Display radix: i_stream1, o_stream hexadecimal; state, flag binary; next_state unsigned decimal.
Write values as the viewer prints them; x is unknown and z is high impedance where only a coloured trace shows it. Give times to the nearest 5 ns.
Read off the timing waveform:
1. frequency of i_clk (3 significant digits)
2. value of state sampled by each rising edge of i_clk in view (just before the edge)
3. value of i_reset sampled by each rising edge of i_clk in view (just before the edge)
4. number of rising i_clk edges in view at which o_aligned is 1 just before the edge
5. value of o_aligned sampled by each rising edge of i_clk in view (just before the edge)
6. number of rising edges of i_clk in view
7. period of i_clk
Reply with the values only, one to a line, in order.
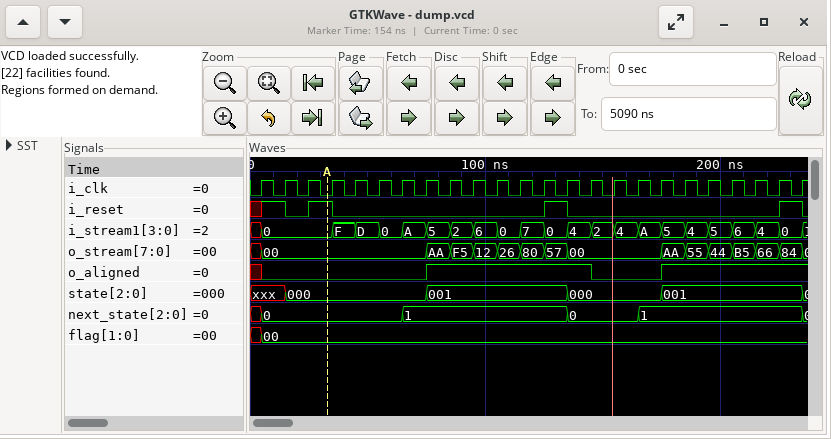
100 MHz
xxx, xxx, 000, 000, 000, 000, 000, 000, 001, 001, 001, 001, 001, 001, 000, 000, 000, 000, 001, 001, 001, 001, 001, 001
x 1 0 1 0 0 0 0 0 0 0 0 0 1 0 0 0 0 0 0 0 0 0 1
13
x 0 0 0 0 0 0 0 1 1 1 1 1 1 1 0 0 0 1 1 1 1 1 1
24
10 ns
